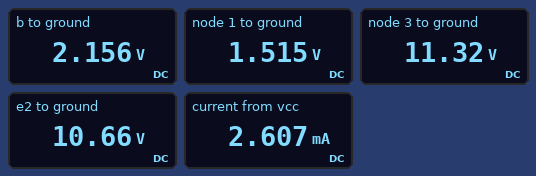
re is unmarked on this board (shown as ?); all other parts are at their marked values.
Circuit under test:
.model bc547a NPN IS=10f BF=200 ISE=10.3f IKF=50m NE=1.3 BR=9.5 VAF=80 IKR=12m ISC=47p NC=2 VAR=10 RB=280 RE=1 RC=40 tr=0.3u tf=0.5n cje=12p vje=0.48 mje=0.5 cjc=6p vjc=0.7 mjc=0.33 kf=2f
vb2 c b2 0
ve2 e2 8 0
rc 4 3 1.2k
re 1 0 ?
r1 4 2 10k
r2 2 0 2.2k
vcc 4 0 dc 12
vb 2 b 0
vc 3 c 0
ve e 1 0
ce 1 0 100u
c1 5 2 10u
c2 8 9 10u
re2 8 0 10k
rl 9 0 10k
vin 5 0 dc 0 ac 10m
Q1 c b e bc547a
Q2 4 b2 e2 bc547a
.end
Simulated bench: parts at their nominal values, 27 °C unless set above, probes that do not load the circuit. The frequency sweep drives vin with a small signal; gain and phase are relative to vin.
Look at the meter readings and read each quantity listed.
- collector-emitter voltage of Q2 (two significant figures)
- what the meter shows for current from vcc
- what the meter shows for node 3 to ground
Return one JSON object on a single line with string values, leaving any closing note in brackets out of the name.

{"collector-emitter voltage of Q2": "1.3 V", "what the meter shows for current from vcc": "2.607 mA", "what the meter shows for node 3 to ground": "11.32 V"}
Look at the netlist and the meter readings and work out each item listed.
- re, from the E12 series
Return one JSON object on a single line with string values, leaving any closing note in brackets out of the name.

{"re, from the E12 series": "2.7 kΩ"}
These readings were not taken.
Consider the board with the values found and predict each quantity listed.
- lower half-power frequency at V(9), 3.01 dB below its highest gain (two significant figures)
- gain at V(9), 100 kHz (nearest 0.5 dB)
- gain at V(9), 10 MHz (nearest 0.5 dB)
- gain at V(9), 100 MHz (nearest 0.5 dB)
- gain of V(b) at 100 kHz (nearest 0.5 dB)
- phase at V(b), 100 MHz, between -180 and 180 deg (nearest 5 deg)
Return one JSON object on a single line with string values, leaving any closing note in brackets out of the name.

{"lower half-power frequency at V(9), 3.01 dB below its highest gain": "37 Hz", "gain at V(9), 100 kHz": "27.5 dB", "gain at V(9), 10 MHz": "19.5 dB", "gain at V(9), 100 MHz": "-8.5 dB", "gain of V(b) at 100 kHz": "0 dB", "phase at V(b), 100 MHz, between -180 and 180 deg": "0 deg"}
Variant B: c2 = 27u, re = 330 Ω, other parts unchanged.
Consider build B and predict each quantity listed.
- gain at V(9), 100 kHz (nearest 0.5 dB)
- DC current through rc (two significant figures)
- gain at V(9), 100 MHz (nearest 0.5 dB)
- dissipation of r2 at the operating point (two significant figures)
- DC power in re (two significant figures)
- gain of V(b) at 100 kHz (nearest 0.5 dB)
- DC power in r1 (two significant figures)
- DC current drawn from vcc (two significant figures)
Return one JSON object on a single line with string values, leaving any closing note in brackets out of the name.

{"gain at V(9), 100 kHz": "41.0 dB", "DC current through rc": "4.2 mA", "gain at V(9), 100 MHz": "-1.0 dB", "dissipation of r2 at the operating point": "2.0 mW", "DC power in re": "5.9 mW", "gain of V(b) at 100 kHz": "0 dB", "DC power in r1": "9.8 mW", "DC current drawn from vcc": "5.8 mA"}
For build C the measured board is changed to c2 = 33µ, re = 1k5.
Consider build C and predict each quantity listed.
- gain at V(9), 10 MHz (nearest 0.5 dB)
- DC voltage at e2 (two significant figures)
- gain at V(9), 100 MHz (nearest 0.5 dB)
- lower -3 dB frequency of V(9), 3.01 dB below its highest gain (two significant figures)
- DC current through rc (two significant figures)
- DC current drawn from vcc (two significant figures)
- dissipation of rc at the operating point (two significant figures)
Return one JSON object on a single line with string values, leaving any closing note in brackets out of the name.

{"gain at V(9), 10 MHz": "21.5 dB", "DC voltage at e2": "10 V", "gain at V(9), 100 MHz": "-5.5 dB", "lower -3 dB frequency of V(9), 3.01 dB below its highest gain": "60 Hz", "DC current through rc": "1.0 mA", "DC current drawn from vcc": "3.0 mA", "dissipation of rc at the operating point": "1.2 mW"}
